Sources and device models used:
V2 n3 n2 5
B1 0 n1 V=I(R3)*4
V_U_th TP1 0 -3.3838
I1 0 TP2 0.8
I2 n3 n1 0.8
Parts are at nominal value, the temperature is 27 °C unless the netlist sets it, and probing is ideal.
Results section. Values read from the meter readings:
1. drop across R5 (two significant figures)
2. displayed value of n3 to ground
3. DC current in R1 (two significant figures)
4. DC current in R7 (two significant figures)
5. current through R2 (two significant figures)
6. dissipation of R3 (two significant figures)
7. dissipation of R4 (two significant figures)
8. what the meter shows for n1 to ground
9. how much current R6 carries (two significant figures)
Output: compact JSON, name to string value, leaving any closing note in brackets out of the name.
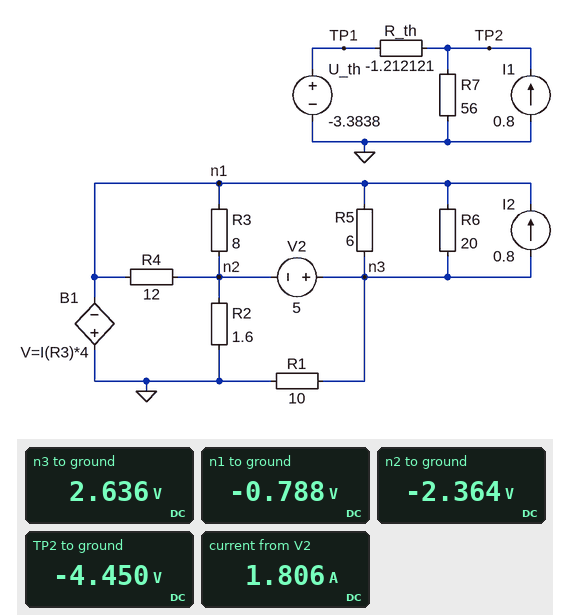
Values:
{"drop across R5": "3.4 V", "displayed value of n3 to ground": "2.636 V", "DC current in R1": "260 mA", "DC current in R7": "79 mA", "current through R2": "1.5 A", "dissipation of R3": "310 mW", "dissipation of R4": "210 mW", "what the meter shows for n1 to ground": "-0.788 V", "how much current R6 carries": "170 mA"}
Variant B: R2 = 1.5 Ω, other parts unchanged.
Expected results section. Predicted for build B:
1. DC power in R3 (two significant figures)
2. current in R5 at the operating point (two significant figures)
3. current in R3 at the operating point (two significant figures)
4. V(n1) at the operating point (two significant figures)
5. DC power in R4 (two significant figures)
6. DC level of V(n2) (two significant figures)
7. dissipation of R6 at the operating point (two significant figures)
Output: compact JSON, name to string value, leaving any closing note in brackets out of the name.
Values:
{"DC power in R3": "290 mW", "current in R5 at the operating point": "580 mA", "current in R3 at the operating point": "190 mA", "V(n1) at the operating point": "-760 mV", "DC power in R4": "190 mW", "DC level of V(n2)": "-2.3 V", "dissipation of R6 at the operating point": "610 mW"}
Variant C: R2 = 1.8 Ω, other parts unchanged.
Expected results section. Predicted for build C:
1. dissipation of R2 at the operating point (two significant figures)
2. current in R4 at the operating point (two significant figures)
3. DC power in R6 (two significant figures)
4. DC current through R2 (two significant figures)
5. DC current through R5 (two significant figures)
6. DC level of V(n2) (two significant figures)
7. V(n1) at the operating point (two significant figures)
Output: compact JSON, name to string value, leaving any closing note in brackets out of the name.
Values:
{"dissipation of R2 at the operating point": "3.6 W", "current in R4 at the operating point": "140 mA", "DC power in R6": "550 mW", "DC current through R2": "1.4 A", "DC current through R5": "550 mA", "DC level of V(n2)": "-2.5 V", "V(n1) at the operating point": "-850 mV"}
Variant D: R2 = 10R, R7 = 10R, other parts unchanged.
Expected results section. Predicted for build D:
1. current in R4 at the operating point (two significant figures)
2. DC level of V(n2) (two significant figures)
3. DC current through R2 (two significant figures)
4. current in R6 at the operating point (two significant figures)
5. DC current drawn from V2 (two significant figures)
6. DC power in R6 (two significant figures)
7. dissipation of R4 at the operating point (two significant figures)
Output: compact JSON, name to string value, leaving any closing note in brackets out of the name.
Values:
{"current in R4 at the operating point": "270 mA", "DC level of V(n2)": "-4.9 V", "DC current through R2": "490 mA", "current in R6 at the operating point": "86 mA", "DC current drawn from V2": "1.2 A", "DC power in R6": "150 mW", "dissipation of R4 at the operating point": "900 mW"}
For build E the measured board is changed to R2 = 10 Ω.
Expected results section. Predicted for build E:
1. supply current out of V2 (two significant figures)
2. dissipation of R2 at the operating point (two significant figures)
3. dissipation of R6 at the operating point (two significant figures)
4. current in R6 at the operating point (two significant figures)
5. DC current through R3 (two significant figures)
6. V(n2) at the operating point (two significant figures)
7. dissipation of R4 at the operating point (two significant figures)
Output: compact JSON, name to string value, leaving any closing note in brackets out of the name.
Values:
{"supply current out of V2": "1.2 A", "dissipation of R2 at the operating point": "2.4 W", "dissipation of R6 at the operating point": "150 mW", "current in R6 at the operating point": "86 mA", "DC current through R3": "410 mA", "V(n2) at the operating point": "-4.9 V", "dissipation of R4 at the operating point": "900 mW"}
